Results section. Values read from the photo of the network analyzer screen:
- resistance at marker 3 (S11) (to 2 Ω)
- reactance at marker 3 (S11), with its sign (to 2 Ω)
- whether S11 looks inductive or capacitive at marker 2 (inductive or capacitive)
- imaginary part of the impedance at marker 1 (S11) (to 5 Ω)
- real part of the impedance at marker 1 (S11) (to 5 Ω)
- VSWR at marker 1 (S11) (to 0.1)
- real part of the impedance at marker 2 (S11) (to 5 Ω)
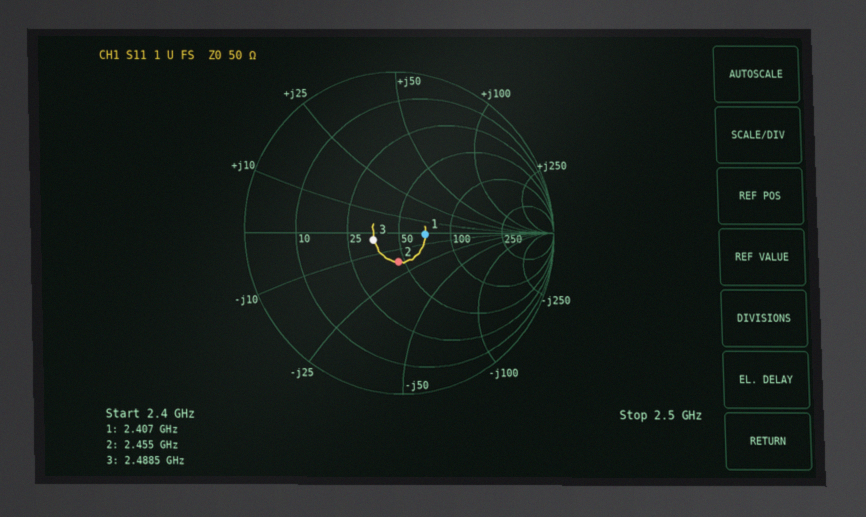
36 Ω
-4 Ω
capacitive
0 Ω
70 Ω
1.4
45 Ω
